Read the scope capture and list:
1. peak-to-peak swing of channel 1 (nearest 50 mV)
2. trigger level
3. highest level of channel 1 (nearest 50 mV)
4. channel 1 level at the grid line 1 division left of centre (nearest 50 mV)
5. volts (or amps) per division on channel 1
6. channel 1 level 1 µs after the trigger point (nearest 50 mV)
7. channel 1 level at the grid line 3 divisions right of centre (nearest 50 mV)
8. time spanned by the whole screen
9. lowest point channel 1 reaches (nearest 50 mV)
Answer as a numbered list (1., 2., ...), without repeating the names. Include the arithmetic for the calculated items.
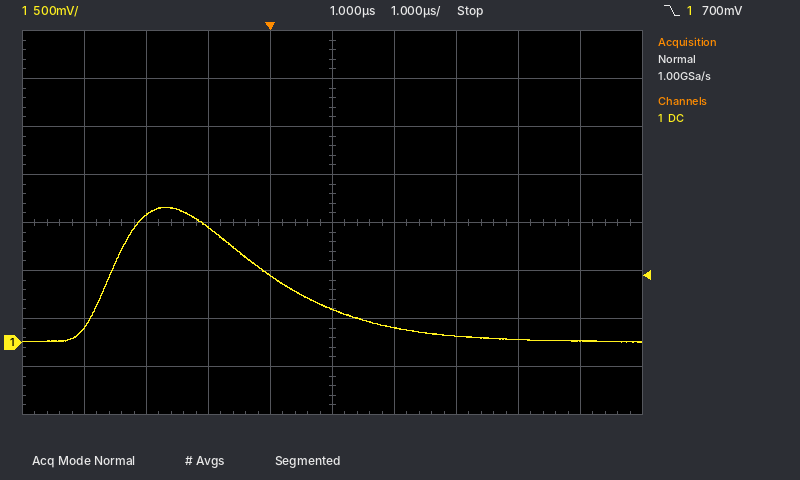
1. 1.40 V − (0 mV) = 1.40 V
2. 700 mV
3. 1.40 V
4. 700 mV
5. 500 mV
6. 350 mV
7. 50 mV
8. 10 µs
9. 0 mV
